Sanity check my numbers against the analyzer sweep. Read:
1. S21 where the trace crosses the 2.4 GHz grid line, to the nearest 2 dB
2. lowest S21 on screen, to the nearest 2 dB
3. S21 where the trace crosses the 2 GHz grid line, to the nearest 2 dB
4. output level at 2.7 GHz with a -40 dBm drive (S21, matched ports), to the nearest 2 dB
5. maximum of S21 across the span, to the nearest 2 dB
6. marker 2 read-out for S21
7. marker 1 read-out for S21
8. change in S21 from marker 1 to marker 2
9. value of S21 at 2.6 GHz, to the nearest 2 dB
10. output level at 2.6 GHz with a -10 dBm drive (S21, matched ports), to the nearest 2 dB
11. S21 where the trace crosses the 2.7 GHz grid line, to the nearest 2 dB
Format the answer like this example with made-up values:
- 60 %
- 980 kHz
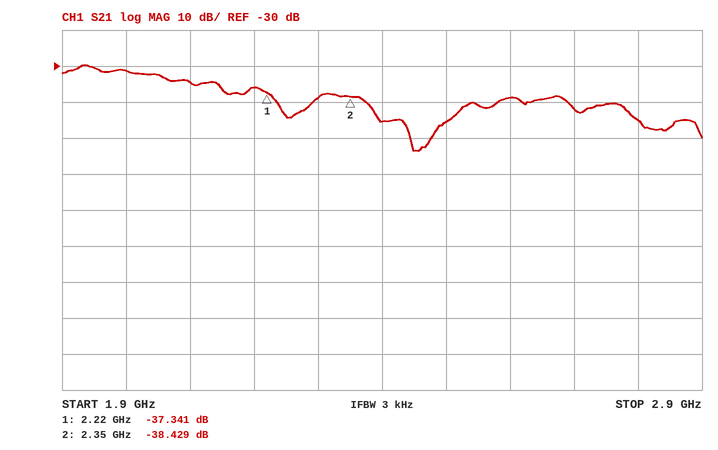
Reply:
- -46 dB
- -54 dB
- -32 dB
- -82 dBm
- -30 dB
- -38.429 dB
- -37.341 dB
- -1.088 dB
- -38 dB
- -48 dBm
- -42 dB
